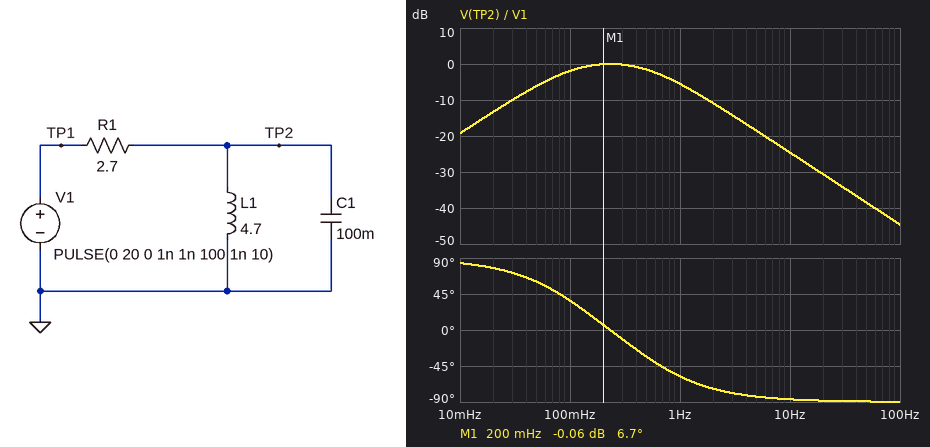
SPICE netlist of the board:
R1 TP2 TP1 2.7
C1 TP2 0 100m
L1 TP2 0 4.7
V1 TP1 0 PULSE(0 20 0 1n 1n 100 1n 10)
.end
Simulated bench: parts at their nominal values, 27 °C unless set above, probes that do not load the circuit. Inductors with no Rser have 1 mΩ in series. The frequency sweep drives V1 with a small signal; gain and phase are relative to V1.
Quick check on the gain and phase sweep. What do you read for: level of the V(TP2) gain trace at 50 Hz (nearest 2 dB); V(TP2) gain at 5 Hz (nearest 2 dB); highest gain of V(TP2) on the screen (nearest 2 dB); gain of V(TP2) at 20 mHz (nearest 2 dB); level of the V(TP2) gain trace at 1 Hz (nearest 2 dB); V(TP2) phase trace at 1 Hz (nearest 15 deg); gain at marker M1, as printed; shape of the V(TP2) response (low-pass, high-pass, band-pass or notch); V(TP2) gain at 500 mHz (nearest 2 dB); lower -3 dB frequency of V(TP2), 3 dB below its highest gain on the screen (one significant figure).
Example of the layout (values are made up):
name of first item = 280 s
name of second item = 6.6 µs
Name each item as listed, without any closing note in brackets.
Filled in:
level of the V(TP2) gain trace at 50 Hz = -38 dB
V(TP2) gain at 5 Hz = -18 dB
highest gain of V(TP2) on the screen = 0 dB
gain of V(TP2) at 20 mHz = -14 dB
level of the V(TP2) gain trace at 1 Hz = -6 dB
V(TP2) phase trace at 1 Hz = -60 deg
gain at marker M1, as printed = -0.06 dB
shape of the V(TP2) response = band-pass
V(TP2) gain at 500 mHz = -2 dB
lower -3 dB frequency of V(TP2), 3 dB below its highest gain on the screen = 80 mHz
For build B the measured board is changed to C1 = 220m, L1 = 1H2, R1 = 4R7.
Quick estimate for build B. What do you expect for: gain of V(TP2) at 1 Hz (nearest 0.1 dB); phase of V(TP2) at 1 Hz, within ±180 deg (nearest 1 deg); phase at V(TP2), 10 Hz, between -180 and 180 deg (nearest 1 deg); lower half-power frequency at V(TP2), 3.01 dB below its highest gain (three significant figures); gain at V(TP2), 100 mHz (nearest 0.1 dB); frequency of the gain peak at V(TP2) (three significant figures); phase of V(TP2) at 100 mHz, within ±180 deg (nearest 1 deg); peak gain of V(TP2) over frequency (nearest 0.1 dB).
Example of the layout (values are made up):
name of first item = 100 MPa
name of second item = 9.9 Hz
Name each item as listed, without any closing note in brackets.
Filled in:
gain of V(TP2) at 1 Hz = -15.5 dB
phase of V(TP2) at 1 Hz, within ±180 deg = -80 deg
phase at V(TP2), 10 Hz, between -180 and 180 deg = -89 deg
lower half-power frequency at V(TP2), 3.01 dB below its highest gain = 242 mHz
gain at V(TP2), 100 mHz = -15.1 dB
frequency of the gain peak at V(TP2) = 310 mHz
phase of V(TP2) at 100 mHz, within ±180 deg = 80 deg
peak gain of V(TP2) over frequency = 0 dB
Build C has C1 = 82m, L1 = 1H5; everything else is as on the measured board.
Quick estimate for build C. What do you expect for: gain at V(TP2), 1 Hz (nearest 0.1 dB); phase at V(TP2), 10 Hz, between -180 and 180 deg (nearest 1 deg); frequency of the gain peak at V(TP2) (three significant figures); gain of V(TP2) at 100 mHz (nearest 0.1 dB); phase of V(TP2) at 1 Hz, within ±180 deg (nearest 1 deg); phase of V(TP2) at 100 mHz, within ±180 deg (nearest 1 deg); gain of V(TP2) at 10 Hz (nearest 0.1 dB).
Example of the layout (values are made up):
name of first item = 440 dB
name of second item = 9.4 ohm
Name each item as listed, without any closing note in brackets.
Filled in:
gain at V(TP2), 1 Hz = -3.5 dB
phase at V(TP2), 10 Hz, between -180 and 180 deg = -86 deg
frequency of the gain peak at V(TP2) = 454 mHz
gain of V(TP2) at 100 mHz = -9.3 dB
phase of V(TP2) at 1 Hz, within ±180 deg = -48 deg
phase of V(TP2) at 100 mHz, within ±180 deg = 70 deg
gain of V(TP2) at 10 Hz = -22.9 dB
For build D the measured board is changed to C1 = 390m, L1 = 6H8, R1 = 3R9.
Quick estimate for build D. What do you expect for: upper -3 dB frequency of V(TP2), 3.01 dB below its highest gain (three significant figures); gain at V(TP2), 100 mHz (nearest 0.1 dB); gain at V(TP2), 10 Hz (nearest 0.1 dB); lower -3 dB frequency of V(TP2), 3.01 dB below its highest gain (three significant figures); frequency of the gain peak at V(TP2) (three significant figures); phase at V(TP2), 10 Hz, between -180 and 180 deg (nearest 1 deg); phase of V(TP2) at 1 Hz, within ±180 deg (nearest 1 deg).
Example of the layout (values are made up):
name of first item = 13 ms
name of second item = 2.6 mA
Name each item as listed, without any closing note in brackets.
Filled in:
upper -3 dB frequency of V(TP2), 3.01 dB below its highest gain = 163 mHz
gain at V(TP2), 100 mHz = 0 dB
gain at V(TP2), 10 Hz = -39.6 dB
lower -3 dB frequency of V(TP2), 3.01 dB below its highest gain = 58.5 mHz
frequency of the gain peak at V(TP2) = 97.7 mHz
phase at V(TP2), 10 Hz, between -180 and 180 deg = -89 deg
phase of V(TP2) at 1 Hz, within ±180 deg = -84 deg
